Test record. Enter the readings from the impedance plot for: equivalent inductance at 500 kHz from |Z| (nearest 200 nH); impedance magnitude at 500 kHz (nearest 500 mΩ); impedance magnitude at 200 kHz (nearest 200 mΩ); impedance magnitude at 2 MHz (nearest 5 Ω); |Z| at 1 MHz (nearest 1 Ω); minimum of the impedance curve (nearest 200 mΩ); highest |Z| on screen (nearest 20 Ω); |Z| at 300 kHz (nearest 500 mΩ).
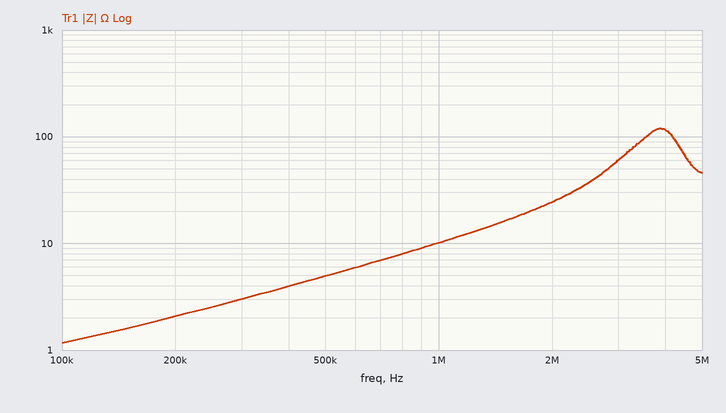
1.6 µH
5.0 Ω
2.0 Ω
25 Ω
10 Ω
1.2 Ω
120 Ω
3.0 Ω
